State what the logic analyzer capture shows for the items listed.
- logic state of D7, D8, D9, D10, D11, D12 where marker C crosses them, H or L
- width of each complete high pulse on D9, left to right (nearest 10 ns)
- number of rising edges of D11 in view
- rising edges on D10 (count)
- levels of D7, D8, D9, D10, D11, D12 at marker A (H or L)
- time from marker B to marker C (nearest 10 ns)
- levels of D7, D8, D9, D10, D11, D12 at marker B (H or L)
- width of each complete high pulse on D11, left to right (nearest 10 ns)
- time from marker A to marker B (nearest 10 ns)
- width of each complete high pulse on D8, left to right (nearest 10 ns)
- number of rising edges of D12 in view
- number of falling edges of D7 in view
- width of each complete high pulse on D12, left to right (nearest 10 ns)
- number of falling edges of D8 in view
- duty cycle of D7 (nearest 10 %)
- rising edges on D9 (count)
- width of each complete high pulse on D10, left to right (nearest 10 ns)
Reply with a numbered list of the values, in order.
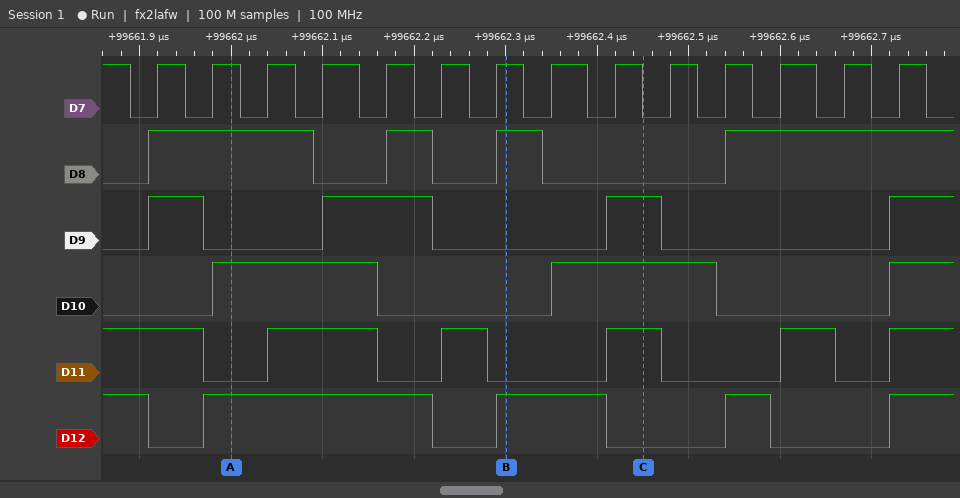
1. D7=L, D8=L, D9=H, D10=H, D11=H, D12=L
2. 60 ns, 120 ns, 60 ns
3. 5
4. 3
5. D7=H, D8=H, D9=L, D10=H, D11=L, D12=H
6. 150 ns
7. D7=H, D8=H, D9=L, D10=L, D11=L, D12=H
8. 120 ns, 50 ns, 60 ns, 60 ns
9. 300 ns
10. 180 ns, 50 ns, 50 ns
11. 4
12. 15
13. 250 ns, 120 ns, 50 ns
14. 3
15. 50 %
16. 4
17. 180 ns, 180 ns
